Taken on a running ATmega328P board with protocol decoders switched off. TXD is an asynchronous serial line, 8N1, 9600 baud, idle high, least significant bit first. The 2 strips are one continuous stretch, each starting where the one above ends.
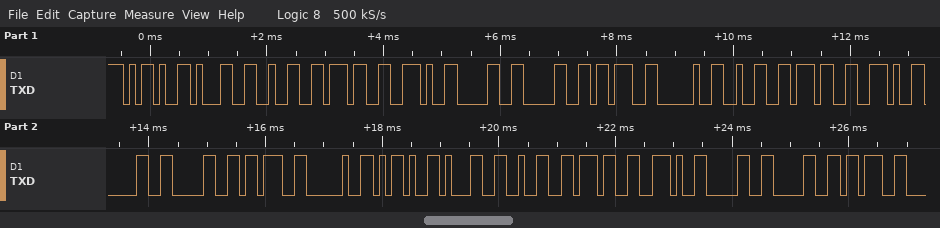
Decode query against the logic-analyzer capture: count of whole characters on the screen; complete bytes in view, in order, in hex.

24
0x2D 0x31 0x32 0x37 0x2E 0x30 0x30 0x3B 0x20 0x32 0x37 0x2E 0x30 0x30 0x3B 0x20 0x2D 0x31 0x32 0x37 0x2E 0x30 0x30 0x3B
